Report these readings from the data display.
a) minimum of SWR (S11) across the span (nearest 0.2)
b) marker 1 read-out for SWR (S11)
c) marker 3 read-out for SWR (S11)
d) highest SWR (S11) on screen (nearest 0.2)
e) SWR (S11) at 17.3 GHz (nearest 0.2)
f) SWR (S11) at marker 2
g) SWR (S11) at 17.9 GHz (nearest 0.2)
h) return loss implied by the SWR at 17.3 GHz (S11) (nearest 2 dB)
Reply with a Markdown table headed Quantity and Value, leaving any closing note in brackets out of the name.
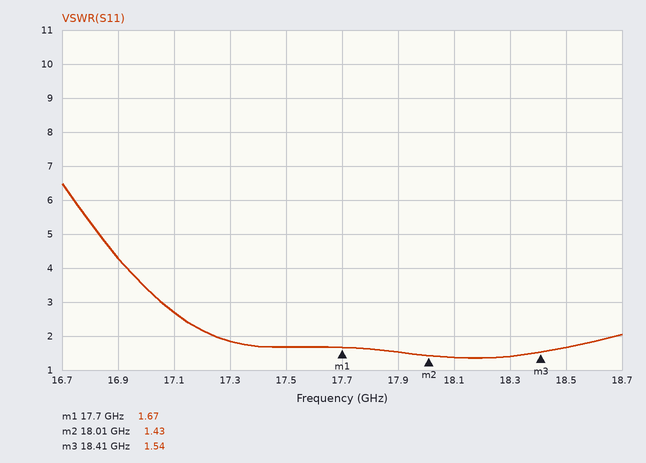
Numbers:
| Quantity | Value |
|---|---|
| minimum of SWR (S11) across the span | 1.4 |
| marker 1 read-out for SWR | 1.67 |
| marker 3 read-out for SWR | 1.54 |
| highest SWR (S11) on screen | 6.4 |
| SWR (S11) at 17.3 GHz | 1.8 |
| SWR (S11) at marker 2 | 1.43 |
| SWR (S11) at 17.9 GHz | 1.6 |
| return loss implied by the SWR at 17.3 GHz (S11) | 10 dB |
